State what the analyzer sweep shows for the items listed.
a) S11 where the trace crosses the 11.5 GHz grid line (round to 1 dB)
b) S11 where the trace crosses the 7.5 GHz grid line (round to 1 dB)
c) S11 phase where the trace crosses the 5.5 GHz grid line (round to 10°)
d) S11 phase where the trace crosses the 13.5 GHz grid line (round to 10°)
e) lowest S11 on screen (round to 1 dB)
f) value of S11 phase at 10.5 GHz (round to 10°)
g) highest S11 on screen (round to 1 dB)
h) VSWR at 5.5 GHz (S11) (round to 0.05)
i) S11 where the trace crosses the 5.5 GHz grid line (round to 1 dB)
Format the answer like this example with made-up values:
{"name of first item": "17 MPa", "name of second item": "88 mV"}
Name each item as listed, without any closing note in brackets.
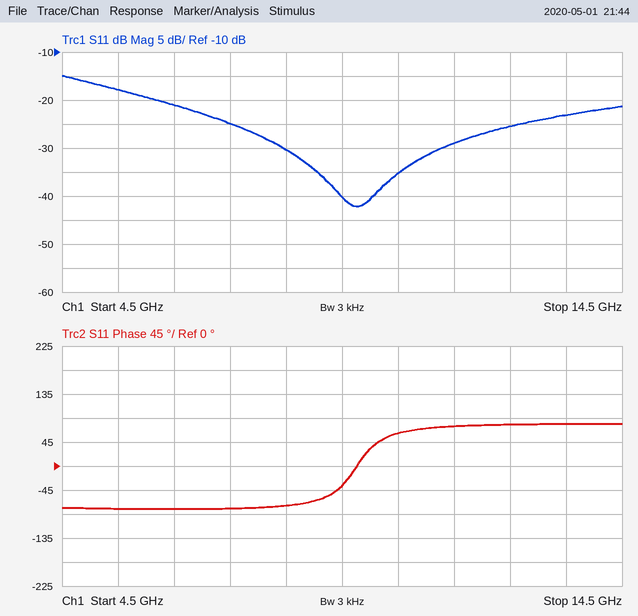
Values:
{"S11 where the trace crosses the 11.5 GHz grid line": "-29 dB", "S11 where the trace crosses the 7.5 GHz grid line": "-25 dB", "S11 phase where the trace crosses the 5.5 GHz grid line": "-80°", "S11 phase where the trace crosses the 13.5 GHz grid line": "80°", "lowest S11 on screen": "-42 dB", "value of S11 phase at 10.5 GHz": "60°", "highest S11 on screen": "-15 dB", "VSWR at 5.5 GHz (S11)": "1.30", "S11 where the trace crosses the 5.5 GHz grid line": "-18 dB"}
